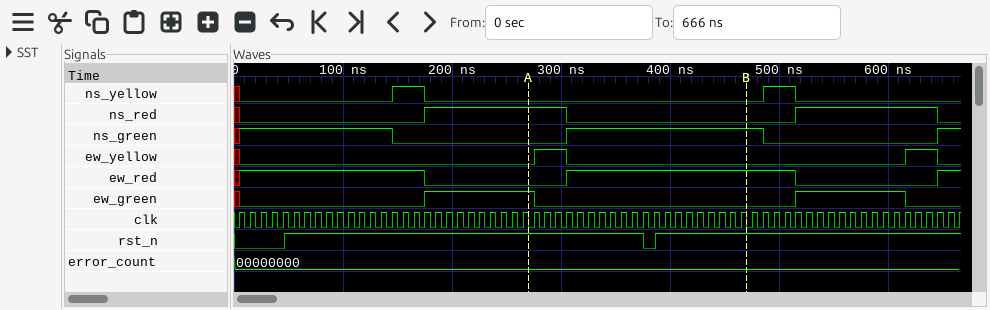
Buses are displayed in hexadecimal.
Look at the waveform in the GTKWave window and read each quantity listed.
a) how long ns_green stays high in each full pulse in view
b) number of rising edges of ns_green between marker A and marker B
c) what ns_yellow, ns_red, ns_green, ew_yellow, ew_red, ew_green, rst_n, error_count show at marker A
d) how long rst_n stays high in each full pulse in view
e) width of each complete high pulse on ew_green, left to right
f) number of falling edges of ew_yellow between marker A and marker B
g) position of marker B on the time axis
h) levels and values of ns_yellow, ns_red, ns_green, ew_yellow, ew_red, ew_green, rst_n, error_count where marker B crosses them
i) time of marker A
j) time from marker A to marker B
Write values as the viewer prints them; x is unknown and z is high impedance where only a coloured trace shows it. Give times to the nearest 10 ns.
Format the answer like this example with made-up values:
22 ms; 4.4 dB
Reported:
180 ns; 1; ns_yellow=0, ns_red=1, ns_green=0, ew_yellow=0, ew_red=0, ew_green=1, rst_n=1, error_count=00000000; 330 ns; 100 ns, 100 ns; 1; 470 ns; ns_yellow=0, ns_red=0, ns_green=1, ew_yellow=0, ew_red=1, ew_green=0, rst_n=1, error_count=00000000; 270 ns; 200 ns
